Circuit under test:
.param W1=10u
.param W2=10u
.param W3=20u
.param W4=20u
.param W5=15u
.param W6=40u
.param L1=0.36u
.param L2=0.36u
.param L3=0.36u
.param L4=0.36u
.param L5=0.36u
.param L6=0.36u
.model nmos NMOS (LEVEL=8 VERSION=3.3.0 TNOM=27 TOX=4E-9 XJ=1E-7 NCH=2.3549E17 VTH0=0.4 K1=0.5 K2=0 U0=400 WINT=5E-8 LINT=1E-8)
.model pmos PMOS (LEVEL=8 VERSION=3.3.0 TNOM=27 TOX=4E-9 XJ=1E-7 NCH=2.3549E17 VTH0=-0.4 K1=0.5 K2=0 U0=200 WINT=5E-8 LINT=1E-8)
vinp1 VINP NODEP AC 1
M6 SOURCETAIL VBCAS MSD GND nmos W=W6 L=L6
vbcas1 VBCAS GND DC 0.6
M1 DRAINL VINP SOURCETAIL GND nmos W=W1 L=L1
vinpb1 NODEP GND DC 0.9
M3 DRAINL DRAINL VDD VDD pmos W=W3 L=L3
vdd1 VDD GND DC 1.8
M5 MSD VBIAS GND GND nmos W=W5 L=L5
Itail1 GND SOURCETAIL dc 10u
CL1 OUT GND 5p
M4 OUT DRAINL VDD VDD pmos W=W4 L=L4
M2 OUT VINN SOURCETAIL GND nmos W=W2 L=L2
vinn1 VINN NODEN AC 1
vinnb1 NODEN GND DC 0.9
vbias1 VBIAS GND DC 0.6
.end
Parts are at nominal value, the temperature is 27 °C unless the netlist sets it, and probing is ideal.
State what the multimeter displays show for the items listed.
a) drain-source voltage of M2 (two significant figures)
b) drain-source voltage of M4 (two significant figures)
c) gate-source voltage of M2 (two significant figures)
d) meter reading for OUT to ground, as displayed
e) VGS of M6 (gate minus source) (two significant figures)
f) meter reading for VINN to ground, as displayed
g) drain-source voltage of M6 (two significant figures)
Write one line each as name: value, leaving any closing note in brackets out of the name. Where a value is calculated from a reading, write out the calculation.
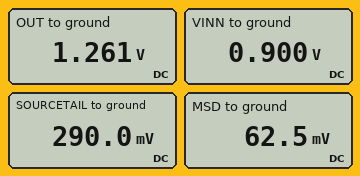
drain-source voltage of M2: 1.261 V - 290 mV = 970 mV
drain-source voltage of M4: 1.261 V - 1.8 V = -540 mV
gate-source voltage of M2: 900 mV - 290 mV = 610 mV
meter reading for OUT to ground, as displayed: 1.261 V
VGS of M6 (gate minus source): 600 mV - 62.5 mV = 540 mV
meter reading for VINN to ground, as displayed: 0.900 V
drain-source voltage of M6: 290 mV - 62.5 mV = 230 mV
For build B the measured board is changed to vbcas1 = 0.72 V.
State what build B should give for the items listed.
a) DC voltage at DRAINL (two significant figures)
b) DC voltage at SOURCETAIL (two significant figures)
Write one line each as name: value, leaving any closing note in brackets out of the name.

DC voltage at DRAINL: 1.2 V
DC voltage at SOURCETAIL: 270 mV
